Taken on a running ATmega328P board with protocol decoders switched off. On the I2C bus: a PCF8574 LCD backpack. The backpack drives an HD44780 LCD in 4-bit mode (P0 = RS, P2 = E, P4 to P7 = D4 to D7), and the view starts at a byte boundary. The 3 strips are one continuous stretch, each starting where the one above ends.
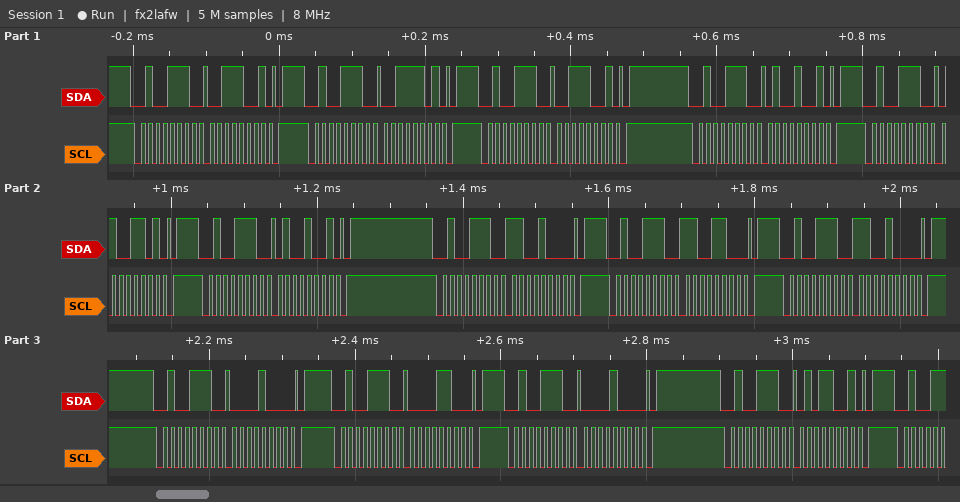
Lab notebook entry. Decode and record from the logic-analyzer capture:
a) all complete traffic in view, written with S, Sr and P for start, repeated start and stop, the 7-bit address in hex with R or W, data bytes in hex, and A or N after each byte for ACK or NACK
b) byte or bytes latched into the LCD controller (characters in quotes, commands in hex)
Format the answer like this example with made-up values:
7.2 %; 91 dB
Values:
S 27W A 39 A P S 27W A 3D A P S 27W A 39 A P S 27W A 49 A P S 27W A 4D A P S 27W A 49 A P S 27W A C8 A P S 27W A CC A P S 27W A C8 A P S 27W A 08 A P S 27W A 0C A P S 27W A 08 A P S 27W A 59 A P; '4' 0xC0
